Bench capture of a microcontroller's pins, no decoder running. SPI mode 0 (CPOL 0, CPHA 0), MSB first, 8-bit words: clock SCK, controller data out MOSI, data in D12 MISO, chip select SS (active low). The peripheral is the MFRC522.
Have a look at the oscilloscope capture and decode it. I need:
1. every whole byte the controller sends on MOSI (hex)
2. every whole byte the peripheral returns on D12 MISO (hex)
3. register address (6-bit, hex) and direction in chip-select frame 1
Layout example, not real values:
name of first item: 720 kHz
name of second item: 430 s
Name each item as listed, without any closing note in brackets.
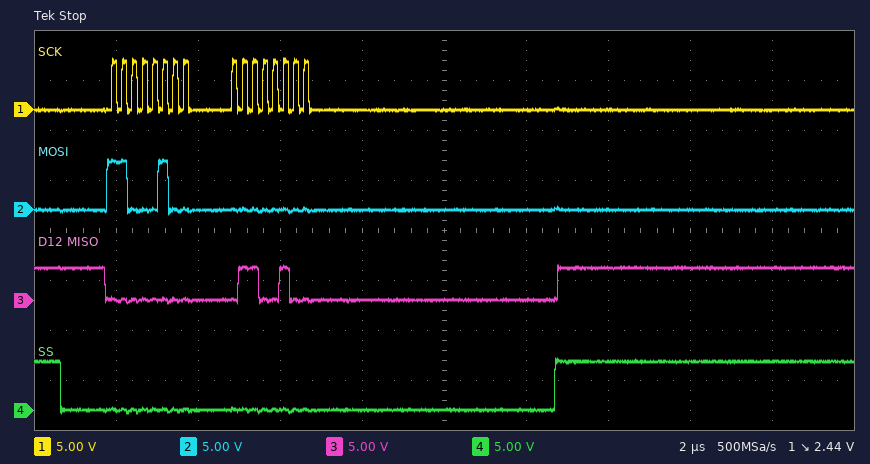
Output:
every whole byte the controller sends on MOSI: C4 00
every whole byte the peripheral returns on D12 MISO: 00 64
register address (6-bit, hex) and direction in chip-select frame 1: 0x22 read
